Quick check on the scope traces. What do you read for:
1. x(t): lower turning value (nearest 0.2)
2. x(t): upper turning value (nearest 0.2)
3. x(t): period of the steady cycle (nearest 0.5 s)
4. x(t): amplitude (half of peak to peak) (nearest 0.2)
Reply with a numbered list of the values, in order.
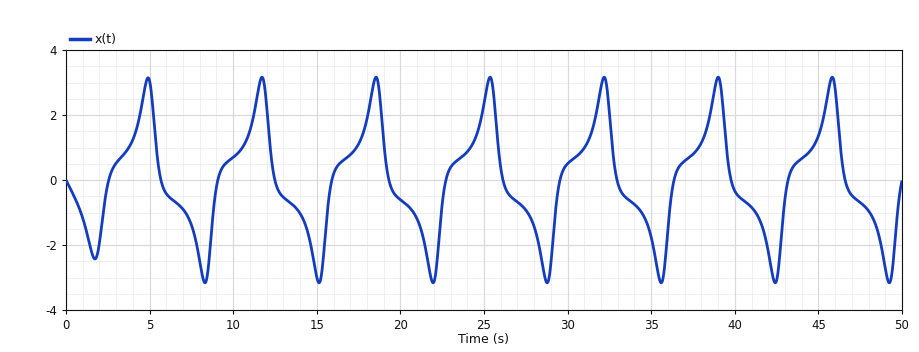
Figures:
1. -3.2
2. 3.2
3. 7.0 s
4. 3.2
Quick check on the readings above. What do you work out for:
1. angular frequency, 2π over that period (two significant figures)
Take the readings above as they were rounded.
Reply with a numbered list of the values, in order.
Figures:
1. 0.90 rad/s
